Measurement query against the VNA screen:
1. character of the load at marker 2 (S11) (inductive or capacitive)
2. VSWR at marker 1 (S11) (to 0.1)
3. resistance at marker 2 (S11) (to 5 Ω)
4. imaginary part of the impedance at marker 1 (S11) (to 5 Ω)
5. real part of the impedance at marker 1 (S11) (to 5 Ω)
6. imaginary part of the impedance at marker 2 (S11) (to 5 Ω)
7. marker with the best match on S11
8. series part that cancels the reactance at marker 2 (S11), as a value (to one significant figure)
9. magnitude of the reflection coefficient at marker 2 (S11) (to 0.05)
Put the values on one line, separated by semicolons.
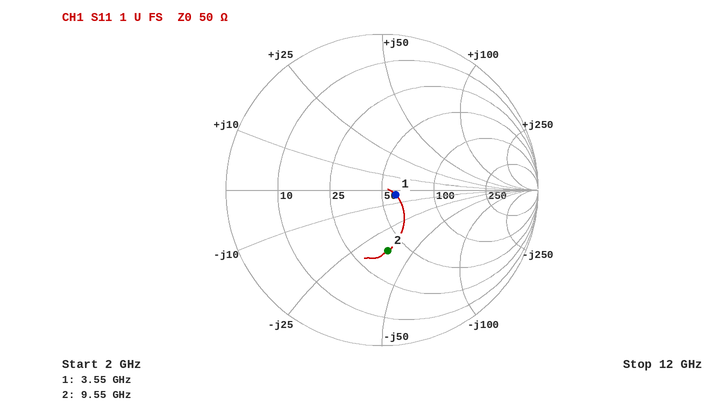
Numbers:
capacitive; 1.2; 40 Ω; -5 Ω; 60 Ω; -35 Ω; marker 1; 600 pH; 0.40
